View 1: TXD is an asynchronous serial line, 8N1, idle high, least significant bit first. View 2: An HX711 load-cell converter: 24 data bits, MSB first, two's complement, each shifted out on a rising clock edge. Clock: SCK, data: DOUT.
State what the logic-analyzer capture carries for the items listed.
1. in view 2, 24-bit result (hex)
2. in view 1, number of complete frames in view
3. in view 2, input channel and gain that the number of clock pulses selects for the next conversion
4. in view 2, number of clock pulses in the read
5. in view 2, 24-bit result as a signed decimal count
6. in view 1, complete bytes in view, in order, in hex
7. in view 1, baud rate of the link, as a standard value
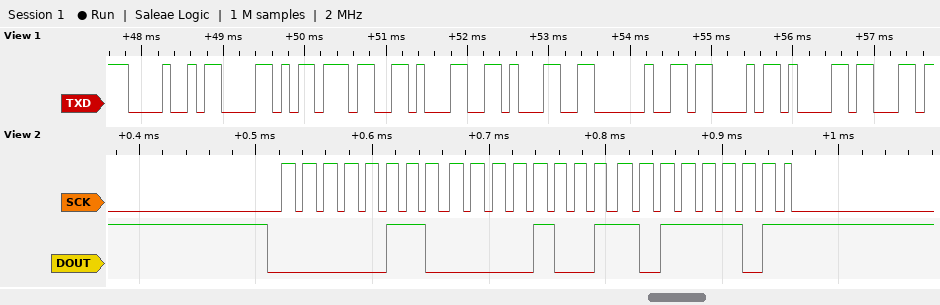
0x0609BD
8
channel A, gain 128
25
395709
48 58 37 31 31 20 43 61
9600 baud
